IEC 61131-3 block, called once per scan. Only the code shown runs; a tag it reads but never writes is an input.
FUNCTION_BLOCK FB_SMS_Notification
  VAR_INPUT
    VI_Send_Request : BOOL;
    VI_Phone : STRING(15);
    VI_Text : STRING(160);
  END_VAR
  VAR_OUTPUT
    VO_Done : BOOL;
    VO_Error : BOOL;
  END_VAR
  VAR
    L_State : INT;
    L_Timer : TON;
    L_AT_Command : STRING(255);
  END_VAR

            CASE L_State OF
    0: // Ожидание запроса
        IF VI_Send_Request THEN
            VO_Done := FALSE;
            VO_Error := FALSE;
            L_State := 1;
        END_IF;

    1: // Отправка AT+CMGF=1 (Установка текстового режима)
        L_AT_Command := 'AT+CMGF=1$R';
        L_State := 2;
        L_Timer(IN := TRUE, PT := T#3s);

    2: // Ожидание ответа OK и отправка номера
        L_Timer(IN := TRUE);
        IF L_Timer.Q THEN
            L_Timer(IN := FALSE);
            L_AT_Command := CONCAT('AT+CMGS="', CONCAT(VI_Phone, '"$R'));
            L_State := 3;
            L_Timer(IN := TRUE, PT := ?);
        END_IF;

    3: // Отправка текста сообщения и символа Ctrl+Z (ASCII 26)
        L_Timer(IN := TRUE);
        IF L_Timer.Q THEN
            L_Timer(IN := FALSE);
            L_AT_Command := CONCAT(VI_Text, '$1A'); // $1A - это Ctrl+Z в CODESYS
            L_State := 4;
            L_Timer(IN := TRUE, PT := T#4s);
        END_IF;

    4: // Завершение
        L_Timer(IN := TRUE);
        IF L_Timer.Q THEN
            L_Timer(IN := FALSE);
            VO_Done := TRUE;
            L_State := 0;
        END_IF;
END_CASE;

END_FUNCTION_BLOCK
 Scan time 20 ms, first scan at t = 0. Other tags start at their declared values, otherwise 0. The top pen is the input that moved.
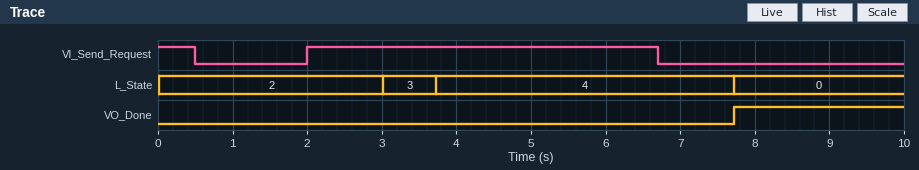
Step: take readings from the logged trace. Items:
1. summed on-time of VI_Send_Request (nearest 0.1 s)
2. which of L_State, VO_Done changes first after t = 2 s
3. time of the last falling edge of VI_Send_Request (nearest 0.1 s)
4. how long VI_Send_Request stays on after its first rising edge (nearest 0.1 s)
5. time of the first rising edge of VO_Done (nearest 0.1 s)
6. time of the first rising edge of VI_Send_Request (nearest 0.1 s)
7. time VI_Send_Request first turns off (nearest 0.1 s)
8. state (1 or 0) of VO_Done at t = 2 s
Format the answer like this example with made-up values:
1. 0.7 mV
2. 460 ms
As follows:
1. 5.2 s
2. L_State
3. 6.7 s
4. 4.7 s
5. 7.7 s
6. 2.0 s
7. 0.5 s
8. 0
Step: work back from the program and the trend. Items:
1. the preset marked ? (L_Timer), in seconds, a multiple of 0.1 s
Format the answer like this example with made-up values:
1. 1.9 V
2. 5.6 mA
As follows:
1. 0.7 s
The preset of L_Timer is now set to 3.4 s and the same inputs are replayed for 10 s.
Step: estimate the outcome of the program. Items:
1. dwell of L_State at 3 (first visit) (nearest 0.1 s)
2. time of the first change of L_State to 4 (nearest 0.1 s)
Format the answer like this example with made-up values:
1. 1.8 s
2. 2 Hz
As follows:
1. 3.4 s
2. 6.4 s
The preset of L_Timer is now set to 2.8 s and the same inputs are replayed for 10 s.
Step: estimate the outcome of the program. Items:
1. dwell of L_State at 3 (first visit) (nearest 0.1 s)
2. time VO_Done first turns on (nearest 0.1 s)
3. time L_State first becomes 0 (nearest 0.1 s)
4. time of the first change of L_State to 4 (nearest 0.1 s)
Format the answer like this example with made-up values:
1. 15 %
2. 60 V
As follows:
1. 2.8 s
2. 9.8 s
3. 9.8 s
4. 5.8 s
